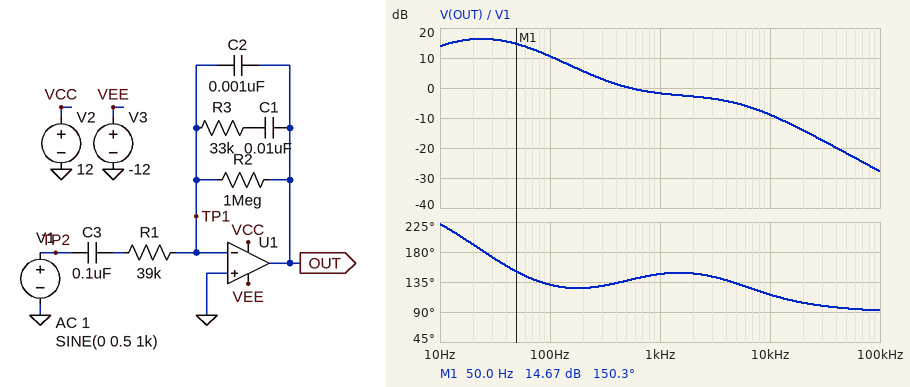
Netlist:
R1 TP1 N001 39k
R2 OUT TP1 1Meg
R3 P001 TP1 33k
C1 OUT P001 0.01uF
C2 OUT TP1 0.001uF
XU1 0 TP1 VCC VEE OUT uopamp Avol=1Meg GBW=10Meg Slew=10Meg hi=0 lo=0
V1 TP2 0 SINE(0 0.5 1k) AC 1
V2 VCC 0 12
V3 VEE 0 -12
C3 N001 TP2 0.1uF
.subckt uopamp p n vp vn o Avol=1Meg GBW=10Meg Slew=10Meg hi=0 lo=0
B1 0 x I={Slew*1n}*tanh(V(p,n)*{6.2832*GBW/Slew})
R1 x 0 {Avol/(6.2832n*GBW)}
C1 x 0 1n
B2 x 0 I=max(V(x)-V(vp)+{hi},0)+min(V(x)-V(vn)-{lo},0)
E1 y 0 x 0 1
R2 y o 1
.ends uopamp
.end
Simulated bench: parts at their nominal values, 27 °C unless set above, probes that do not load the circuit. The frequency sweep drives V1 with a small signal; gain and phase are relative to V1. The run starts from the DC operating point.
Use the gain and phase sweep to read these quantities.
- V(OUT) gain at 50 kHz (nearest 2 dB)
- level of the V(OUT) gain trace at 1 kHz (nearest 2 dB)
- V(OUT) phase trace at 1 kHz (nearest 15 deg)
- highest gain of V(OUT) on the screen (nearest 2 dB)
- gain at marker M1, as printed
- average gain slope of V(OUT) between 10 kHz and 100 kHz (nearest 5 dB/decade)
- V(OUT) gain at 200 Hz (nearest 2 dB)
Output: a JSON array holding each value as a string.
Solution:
["-22 dB", "-2 dB", "150 deg", "16 dB", "14.67 dB", "-20 dB/decade", "6 dB"]
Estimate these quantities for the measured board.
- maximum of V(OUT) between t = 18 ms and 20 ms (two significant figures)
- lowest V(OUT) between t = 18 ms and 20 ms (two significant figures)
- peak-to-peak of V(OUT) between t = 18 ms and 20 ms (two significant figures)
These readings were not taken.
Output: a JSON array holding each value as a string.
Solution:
["420 mV", "-390 mV", "820 mV"]
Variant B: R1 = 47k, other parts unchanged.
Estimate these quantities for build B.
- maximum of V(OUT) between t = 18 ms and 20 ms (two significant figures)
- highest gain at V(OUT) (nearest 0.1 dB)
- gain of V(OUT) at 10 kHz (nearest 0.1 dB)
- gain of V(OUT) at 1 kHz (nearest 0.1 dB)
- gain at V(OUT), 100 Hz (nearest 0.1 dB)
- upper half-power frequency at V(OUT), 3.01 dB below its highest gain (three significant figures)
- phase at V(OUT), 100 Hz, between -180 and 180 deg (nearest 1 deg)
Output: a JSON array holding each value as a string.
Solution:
["350 mV", "15.9 dB", "-10.5 dB", "-3.4 dB", "9.2 dB", "56.9 Hz", "127 deg"]
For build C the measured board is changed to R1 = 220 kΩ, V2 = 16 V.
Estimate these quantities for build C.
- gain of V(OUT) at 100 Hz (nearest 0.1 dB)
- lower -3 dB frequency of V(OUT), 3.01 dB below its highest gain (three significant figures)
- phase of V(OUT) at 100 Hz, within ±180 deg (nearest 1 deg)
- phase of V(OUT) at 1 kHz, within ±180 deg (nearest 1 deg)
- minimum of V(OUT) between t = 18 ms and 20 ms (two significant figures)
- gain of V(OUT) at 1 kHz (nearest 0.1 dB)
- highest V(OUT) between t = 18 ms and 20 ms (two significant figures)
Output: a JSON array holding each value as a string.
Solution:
["-3.8 dB", "4.02 Hz", "113 deg", "145 deg", "-71 mV", "-16.8 dB", "75 mV"]
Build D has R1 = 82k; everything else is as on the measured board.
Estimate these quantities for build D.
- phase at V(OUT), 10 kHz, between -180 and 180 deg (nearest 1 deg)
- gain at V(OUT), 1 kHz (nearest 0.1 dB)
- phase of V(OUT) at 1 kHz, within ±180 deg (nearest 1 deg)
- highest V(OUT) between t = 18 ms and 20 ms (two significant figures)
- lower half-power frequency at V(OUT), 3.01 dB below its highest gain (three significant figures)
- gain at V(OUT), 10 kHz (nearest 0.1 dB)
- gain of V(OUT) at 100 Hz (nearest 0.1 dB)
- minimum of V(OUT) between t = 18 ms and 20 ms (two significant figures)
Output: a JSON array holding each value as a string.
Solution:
["116 deg", "-8.2 dB", "146 deg", "210 mV", "6.79 Hz", "-15.4 dB", "4.6 dB", "-180 mV"]
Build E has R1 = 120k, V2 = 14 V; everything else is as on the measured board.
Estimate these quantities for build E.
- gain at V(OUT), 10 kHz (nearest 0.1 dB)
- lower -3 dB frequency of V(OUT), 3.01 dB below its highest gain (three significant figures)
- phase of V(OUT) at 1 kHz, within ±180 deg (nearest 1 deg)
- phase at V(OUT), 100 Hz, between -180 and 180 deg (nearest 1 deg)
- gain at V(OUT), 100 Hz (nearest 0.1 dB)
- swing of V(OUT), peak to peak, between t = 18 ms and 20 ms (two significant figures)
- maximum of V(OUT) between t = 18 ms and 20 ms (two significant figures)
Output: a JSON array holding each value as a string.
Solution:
["-18.7 dB", "5.66 Hz", "145 deg", "116 deg", "1.4 dB", "270 mV", "140 mV"]
